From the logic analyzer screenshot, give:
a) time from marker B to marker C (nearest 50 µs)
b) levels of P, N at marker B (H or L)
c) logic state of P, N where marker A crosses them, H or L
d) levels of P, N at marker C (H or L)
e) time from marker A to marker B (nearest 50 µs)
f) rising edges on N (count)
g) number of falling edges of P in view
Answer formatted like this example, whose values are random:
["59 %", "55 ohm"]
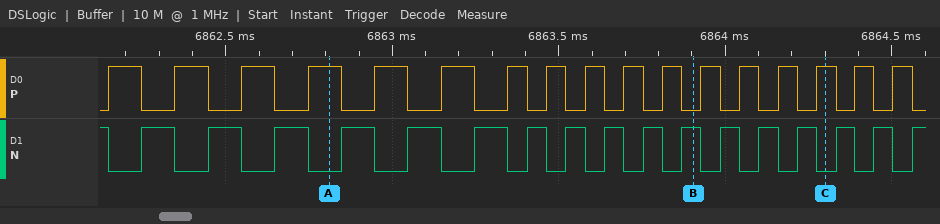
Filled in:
["400 µs", "P=L, N=H", "P=H, N=L", "P=H, N=L", "1100 µs", "17", "17"]
